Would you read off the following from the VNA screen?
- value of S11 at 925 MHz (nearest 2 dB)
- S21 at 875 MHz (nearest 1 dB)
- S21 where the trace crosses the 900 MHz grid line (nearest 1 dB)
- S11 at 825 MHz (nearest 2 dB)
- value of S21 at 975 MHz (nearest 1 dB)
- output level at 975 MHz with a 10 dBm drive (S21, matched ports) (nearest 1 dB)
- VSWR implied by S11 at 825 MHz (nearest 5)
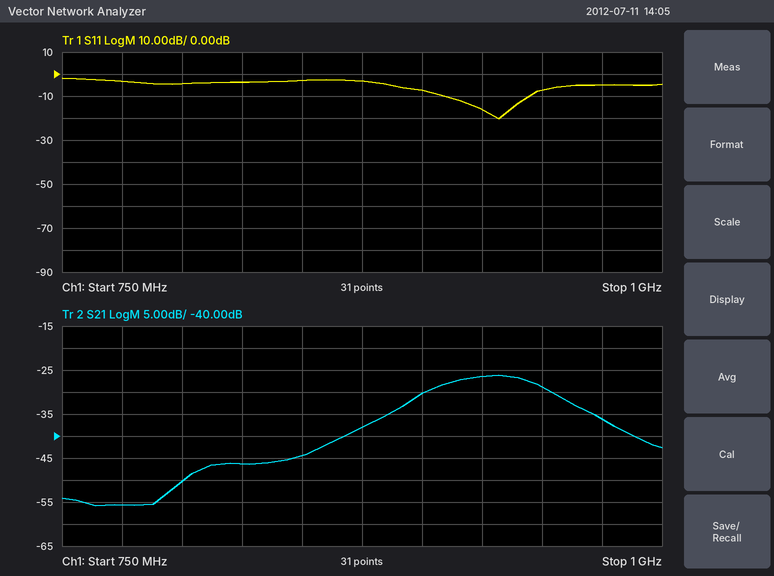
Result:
-16 dB
-38 dB
-30 dB
-4 dB
-36 dB
-26 dBm
5
